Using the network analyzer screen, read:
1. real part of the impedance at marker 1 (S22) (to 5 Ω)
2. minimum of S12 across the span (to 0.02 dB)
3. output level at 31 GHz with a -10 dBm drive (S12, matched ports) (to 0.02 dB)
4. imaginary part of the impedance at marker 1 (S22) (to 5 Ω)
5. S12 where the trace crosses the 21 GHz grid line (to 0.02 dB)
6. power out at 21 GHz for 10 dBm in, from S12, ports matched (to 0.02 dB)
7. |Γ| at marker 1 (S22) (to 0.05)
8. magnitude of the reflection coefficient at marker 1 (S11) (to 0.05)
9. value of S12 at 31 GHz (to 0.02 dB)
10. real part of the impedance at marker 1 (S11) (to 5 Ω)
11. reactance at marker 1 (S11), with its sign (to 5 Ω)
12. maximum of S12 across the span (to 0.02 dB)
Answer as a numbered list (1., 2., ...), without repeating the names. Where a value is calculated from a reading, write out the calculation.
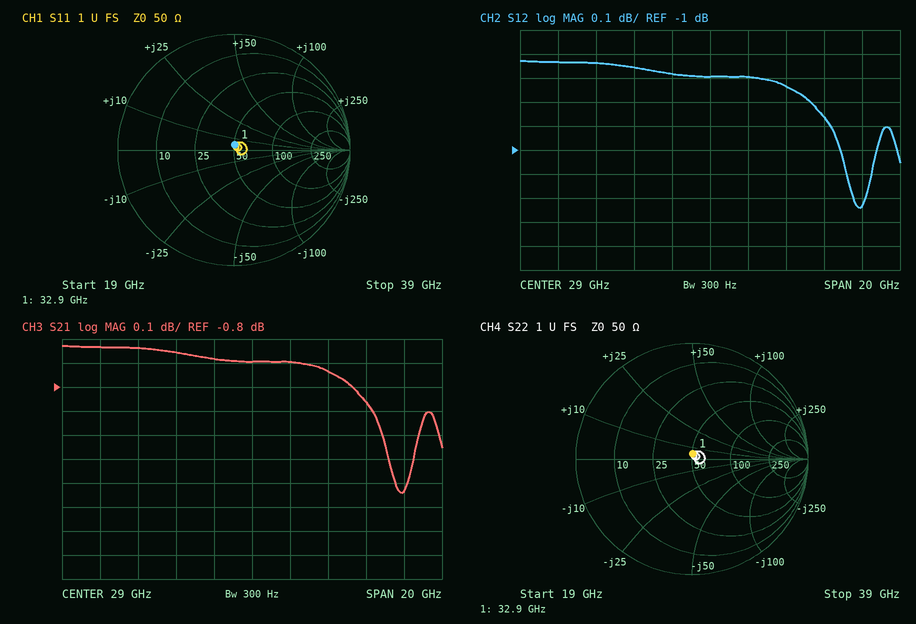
1. 50 Ω
2. -1.24 dB
3. -10 dBm + (-0.70 dB) = -10.70 dBm
4. +5 Ω
5. -0.64 dB
6. 10 dBm + (-0.64 dB) = 9.36 dBm
7. 0.05
8. 0.05
9. -0.70 dB
10. 50 Ω
11. +5 Ω
12. -0.62 dB
